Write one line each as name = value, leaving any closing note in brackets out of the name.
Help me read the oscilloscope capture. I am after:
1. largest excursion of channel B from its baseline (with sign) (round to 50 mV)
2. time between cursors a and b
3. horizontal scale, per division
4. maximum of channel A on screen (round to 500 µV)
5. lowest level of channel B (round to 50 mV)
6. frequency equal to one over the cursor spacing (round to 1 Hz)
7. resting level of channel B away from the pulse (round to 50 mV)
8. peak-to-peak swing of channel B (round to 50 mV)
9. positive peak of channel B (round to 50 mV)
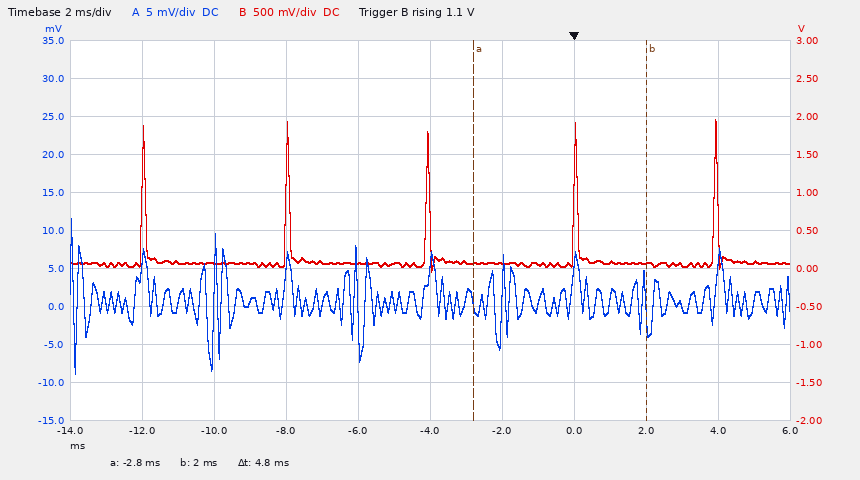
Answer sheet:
largest excursion of channel B from its baseline (with sign) = +1.90 V
time between cursors a and b = 4.8 ms
horizontal scale, per division = 2 ms
maximum of channel A on screen = 11.5 mV
lowest level of channel B = -50 mV
frequency equal to one over the cursor spacing = 208 Hz
resting level of channel B away from the pulse = 50 mV
peak-to-peak swing of channel B = 2.00 V
positive peak of channel B = 1.95 V
